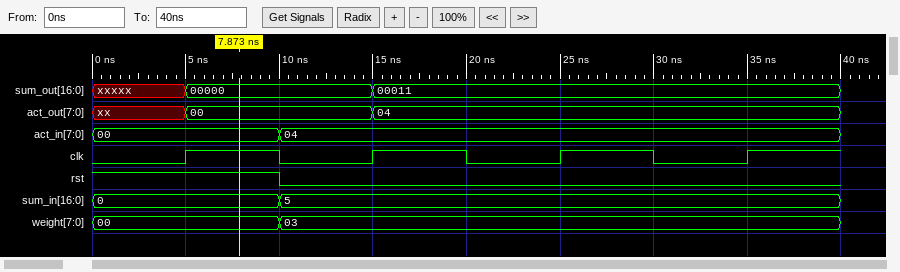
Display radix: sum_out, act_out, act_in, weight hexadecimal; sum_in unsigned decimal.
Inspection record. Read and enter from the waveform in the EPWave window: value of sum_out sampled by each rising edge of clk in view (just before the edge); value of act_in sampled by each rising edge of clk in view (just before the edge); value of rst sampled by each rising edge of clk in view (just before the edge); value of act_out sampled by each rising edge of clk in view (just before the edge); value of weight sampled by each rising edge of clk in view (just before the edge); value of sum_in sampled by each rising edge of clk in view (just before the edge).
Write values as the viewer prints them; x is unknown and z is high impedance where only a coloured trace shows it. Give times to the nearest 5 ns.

xxxxx, 00000, 00011, 00011
00, 04, 04, 04
1 0 0 0
xx, 00, 04, 04
00, 03, 03, 03
0, 5, 5, 5
